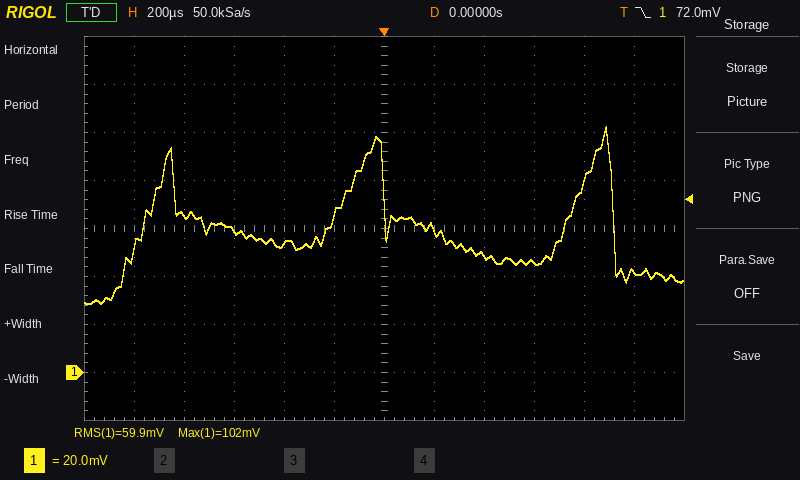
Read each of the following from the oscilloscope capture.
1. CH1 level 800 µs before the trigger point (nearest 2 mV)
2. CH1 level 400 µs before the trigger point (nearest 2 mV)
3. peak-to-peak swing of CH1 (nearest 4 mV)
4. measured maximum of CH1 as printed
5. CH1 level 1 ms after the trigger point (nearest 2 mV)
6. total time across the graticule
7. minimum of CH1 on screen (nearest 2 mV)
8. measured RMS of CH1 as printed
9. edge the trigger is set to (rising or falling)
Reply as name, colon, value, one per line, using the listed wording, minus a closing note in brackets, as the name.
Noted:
CH1 level 800 µs before the trigger point: 66 mV
CH1 level 400 µs before the trigger point: 54 mV
peak-to-peak swing of CH1: 72 mV
measured maximum of CH1 as printed: 102 mV
CH1 level 1 ms after the trigger point: 42 mV
total time across the graticule: 2.4 ms
minimum of CH1 on screen: 28 mV
measured RMS of CH1 as printed: 59.9 mV
edge the trigger is set to: falling
